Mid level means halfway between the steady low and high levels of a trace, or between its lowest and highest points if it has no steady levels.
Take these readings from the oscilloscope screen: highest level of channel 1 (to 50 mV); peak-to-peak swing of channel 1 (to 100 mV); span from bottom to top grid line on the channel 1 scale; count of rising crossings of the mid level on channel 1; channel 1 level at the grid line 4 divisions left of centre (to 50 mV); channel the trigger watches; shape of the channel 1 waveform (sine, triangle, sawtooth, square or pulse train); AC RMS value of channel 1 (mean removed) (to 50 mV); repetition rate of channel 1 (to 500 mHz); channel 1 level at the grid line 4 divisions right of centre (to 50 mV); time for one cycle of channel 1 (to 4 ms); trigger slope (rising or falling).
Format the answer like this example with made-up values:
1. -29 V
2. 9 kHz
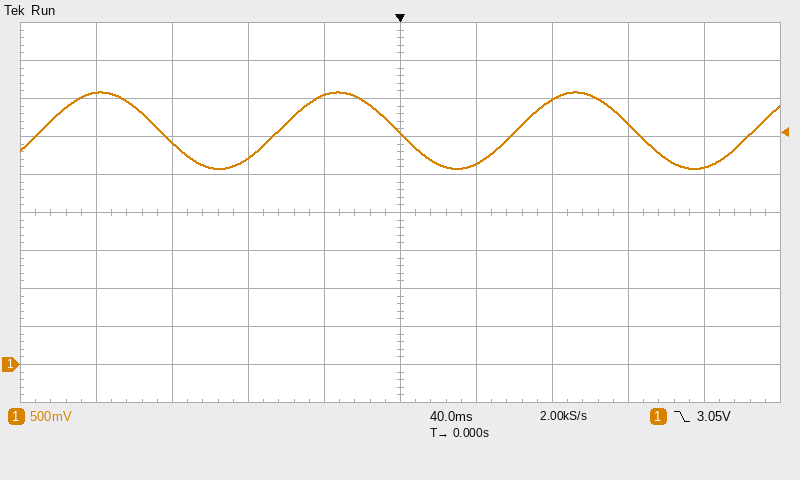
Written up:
1. 3.60 V
2. 1.00 V
3. 5 V
4. 4
5. 3.60 V
6. channel 1
7. sine
8. 350 mV
9. 8.0 Hz
10. 2.60 V
11. 124 ms
12. falling
